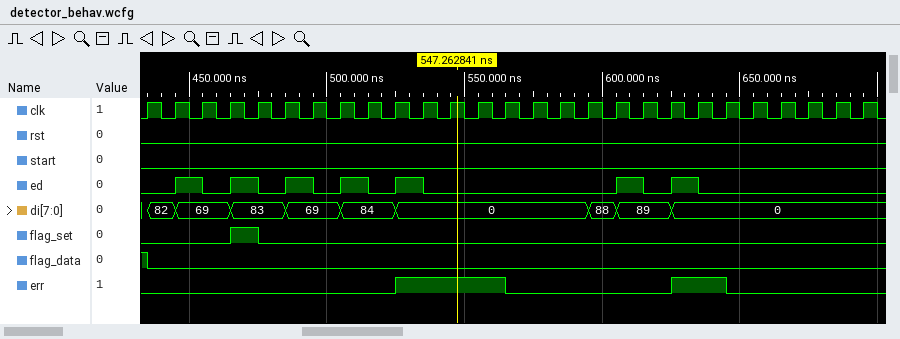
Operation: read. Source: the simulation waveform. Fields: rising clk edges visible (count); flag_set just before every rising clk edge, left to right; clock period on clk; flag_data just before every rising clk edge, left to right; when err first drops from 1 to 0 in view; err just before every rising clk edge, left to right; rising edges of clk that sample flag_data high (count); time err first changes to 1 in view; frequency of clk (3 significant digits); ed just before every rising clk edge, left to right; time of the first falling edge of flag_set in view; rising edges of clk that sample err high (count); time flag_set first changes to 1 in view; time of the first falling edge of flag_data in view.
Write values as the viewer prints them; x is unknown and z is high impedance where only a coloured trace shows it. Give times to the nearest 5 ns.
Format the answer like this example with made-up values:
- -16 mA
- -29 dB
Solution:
- 27
- 0 0 0 0 1 0 0 0 0 0 0 0 0 0 0 0 0 0 0 0 0 0 0 0 0 0 0
- 10 ns
- 1 0 0 0 0 0 0 0 0 0 0 0 0 0 0 0 0 0 0 0 0 0 0 0 0 0 0
- 565 ns
- 0 0 0 0 0 0 0 0 0 0 1 1 1 1 0 0 0 0 0 0 1 1 0 0 0 0 0
- 1
- 525 ns
- 100 MHz
- 0 0 1 0 1 0 1 0 1 0 1 0 0 0 0 0 0 0 1 0 1 0 0 0 0 0 0
- 475 ns
- 6
- 465 ns
- 435 ns
